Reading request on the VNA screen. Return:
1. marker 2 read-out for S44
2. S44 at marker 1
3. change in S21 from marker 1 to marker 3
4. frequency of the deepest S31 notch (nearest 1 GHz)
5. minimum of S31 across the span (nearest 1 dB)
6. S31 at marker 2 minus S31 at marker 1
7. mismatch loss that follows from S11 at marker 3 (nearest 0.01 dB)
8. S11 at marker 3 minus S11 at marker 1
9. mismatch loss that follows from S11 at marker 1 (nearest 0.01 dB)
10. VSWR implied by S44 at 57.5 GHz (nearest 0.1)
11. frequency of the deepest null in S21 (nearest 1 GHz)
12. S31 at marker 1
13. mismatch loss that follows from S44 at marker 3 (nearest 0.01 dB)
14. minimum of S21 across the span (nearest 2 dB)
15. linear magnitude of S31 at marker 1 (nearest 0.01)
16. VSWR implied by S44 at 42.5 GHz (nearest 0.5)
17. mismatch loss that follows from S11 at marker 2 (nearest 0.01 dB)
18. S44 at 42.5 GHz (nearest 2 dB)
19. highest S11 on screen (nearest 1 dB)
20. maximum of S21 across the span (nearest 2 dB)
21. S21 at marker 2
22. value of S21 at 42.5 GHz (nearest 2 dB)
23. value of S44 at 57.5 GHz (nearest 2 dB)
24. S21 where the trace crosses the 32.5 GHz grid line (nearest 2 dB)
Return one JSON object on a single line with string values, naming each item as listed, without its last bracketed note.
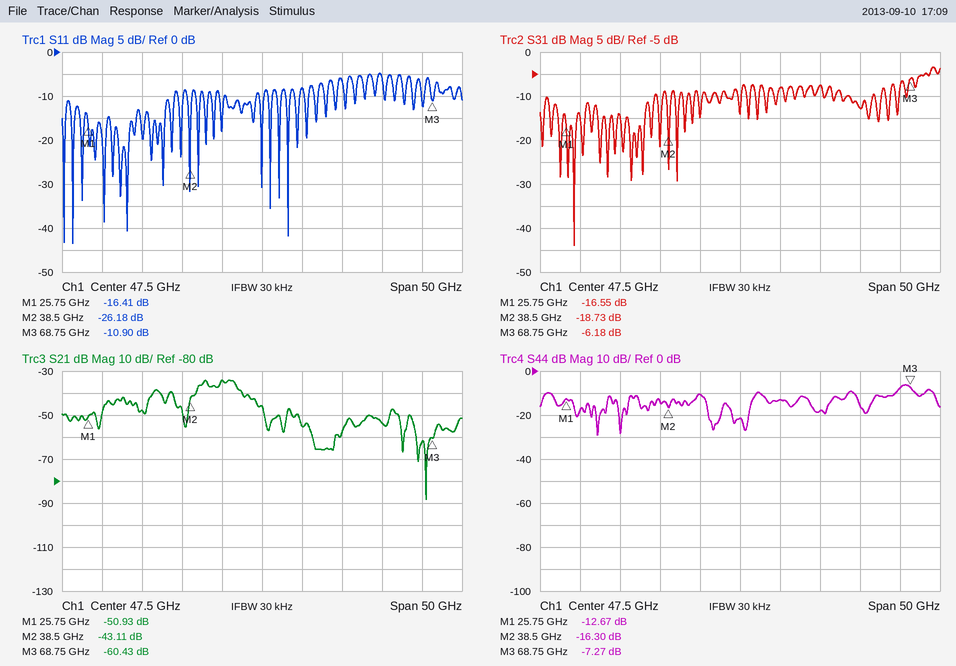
{"marker 2 read-out for S44": "-16.30 dB", "S44 at marker 1": "-12.67 dB", "change in S21 from marker 1 to marker 3": "-9.50 dB", "frequency of the deepest S31 notch": "27 GHz", "minimum of S31 across the span": "-44 dB", "S31 at marker 2 minus S31 at marker 1": "-2.18 dB", "mismatch loss that follows from S11 at marker 3": "0.37 dB", "S11 at marker 3 minus S11 at marker 1": "5.51 dB", "mismatch loss that follows from S11 at marker 1": "0.10 dB", "VSWR implied by S44 at 57.5 GHz": "1.3", "frequency of the deepest null in S21": "68 GHz", "S31 at marker 1": "-16.55 dB", "mismatch loss that follows from S44 at marker 3": "0.90 dB", "minimum of S21 across the span": "-88 dB", "linear magnitude of S31 at marker 1": "0.15", "VSWR implied by S44 at 42.5 GHz": "2.0", "mismatch loss that follows from S11 at marker 2": "0.01 dB", "S44 at 42.5 GHz": "-10 dB", "highest S11 on screen": "-5 dB", "maximum of S21 across the span": "-34 dB", "S21 at marker 2": "-43.11 dB", "value of S21 at 42.5 GHz": "-34 dB", "value of S44 at 57.5 GHz": "-18 dB", "S21 where the trace crosses the 32.5 GHz grid line": "-48 dB"}
